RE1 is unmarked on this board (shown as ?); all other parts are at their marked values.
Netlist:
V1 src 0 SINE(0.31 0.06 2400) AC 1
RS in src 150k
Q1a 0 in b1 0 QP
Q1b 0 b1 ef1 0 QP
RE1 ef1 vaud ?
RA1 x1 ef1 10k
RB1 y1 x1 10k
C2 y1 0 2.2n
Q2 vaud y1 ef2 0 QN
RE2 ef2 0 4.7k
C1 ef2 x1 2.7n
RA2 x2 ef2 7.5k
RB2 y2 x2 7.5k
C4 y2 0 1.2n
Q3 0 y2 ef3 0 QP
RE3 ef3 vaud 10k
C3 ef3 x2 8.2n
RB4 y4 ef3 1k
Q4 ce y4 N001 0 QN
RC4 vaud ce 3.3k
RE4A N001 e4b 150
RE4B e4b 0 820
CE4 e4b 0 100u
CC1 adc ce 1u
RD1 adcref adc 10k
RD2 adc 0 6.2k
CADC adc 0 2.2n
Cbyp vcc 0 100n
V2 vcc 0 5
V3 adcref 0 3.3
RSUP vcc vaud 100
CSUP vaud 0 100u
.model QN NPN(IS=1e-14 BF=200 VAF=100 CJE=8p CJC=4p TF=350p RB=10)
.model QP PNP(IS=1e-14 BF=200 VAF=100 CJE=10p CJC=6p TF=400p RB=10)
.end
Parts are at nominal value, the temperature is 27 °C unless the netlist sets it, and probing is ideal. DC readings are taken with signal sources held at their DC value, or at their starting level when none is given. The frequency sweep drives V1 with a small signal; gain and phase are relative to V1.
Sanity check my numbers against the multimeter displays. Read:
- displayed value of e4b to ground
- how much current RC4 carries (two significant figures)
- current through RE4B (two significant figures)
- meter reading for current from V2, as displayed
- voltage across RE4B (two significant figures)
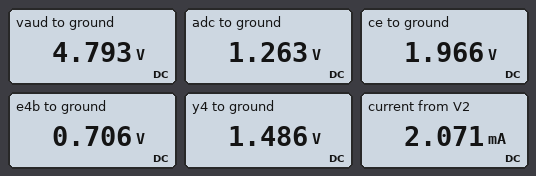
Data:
0.706 V
860 µA
860 µA
2.071 mA
710 mV
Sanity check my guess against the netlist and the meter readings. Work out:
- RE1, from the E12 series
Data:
4.7 kΩ
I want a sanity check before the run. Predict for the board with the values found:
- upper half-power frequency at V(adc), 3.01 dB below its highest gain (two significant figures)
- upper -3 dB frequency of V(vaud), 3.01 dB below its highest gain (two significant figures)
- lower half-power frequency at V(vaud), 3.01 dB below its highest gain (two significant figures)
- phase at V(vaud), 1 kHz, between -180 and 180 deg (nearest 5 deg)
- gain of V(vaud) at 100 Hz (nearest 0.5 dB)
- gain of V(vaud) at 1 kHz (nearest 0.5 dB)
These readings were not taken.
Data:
6.1 kHz
25 Hz
4.4 Hz
65 deg
-27.5 dB
-48.0 dB
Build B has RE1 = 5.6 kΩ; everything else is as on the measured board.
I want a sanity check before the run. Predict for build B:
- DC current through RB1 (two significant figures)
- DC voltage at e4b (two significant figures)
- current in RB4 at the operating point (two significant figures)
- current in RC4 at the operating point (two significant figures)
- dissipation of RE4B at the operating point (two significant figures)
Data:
840 nA
700 mV
4.2 µA
850 µA
600 µW
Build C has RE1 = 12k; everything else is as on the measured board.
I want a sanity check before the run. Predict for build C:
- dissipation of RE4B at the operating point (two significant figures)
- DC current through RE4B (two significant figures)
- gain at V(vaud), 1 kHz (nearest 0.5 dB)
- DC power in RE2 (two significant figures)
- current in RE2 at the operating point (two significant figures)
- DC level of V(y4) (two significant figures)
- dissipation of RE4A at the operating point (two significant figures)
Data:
550 µW
820 µA
-47.5 dB
130 µW
170 µA
1.4 V
100 µW
